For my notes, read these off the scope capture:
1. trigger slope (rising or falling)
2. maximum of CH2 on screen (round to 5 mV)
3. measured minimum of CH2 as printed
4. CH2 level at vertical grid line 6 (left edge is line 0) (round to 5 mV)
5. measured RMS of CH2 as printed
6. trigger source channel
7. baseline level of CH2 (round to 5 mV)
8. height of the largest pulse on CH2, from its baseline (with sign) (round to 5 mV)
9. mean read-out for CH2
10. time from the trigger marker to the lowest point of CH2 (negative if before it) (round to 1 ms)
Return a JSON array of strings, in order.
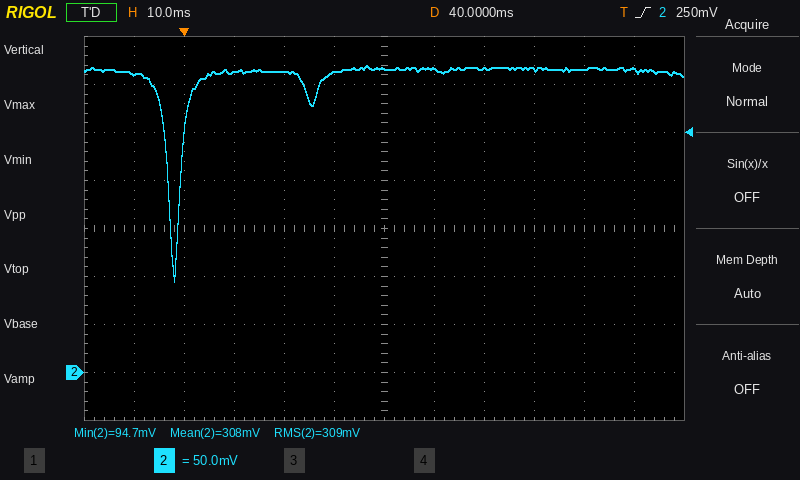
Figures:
["rising", "320 mV", "94.7 mV", "315 mV", "309 mV", "CH2", "315 mV", "-220 mV", "308 mV", "-2 ms"]
